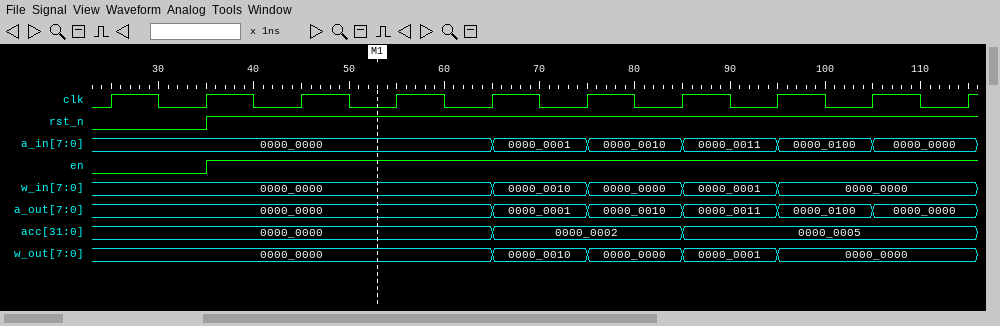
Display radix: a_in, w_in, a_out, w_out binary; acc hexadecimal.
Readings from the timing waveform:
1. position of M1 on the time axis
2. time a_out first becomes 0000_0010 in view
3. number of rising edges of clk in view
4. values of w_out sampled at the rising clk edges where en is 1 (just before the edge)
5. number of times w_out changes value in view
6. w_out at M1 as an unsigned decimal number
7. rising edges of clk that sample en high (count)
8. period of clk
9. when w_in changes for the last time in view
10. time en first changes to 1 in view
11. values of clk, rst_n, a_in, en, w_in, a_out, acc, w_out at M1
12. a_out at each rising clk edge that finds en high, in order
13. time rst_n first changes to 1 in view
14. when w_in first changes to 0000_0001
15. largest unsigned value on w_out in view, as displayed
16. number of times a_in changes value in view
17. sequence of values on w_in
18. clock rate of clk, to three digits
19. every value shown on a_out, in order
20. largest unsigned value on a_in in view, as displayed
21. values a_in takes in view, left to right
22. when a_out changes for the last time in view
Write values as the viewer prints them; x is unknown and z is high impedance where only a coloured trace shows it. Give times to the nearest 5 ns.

55 ns
75 ns
10
0000_0000, 0000_0000, 0000_0000, 0000_0010, 0000_0000, 0000_0001, 0000_0000, 0000_0000
4
0
8
10 ns
95 ns
35 ns
clk=0, rst_n=1, a_in=0000_0000, en=1, w_in=0000_0000, a_out=0000_0000, acc=0000_0000, w_out=0000_0000
0000_0000, 0000_0000, 0000_0000, 0000_0001, 0000_0010, 0000_0011, 0000_0100, 0000_0000
35 ns
85 ns
0000_0010
5
0000_0000, 0000_0010, 0000_0000, 0000_0001, 0000_0000
100 MHz
0000_0000, 0000_0001, 0000_0010, 0000_0011, 0000_0100, 0000_0000
0000_0100
0000_0000, 0000_0001, 0000_0010, 0000_0011, 0000_0100, 0000_0000
105 ns
